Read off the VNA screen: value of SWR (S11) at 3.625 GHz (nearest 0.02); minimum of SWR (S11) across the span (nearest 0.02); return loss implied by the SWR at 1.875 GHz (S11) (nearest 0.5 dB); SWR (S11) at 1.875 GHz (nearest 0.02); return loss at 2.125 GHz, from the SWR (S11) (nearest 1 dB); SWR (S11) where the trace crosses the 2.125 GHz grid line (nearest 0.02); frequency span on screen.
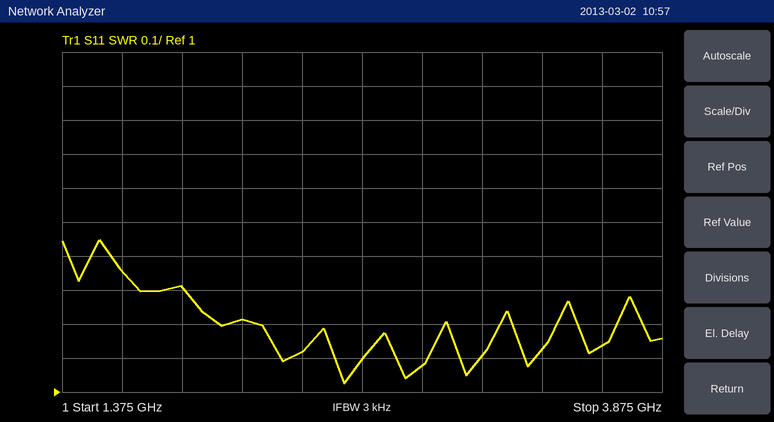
1.14
1.02
17.5 dB
1.30
20 dB
1.22
2.5 GHz
